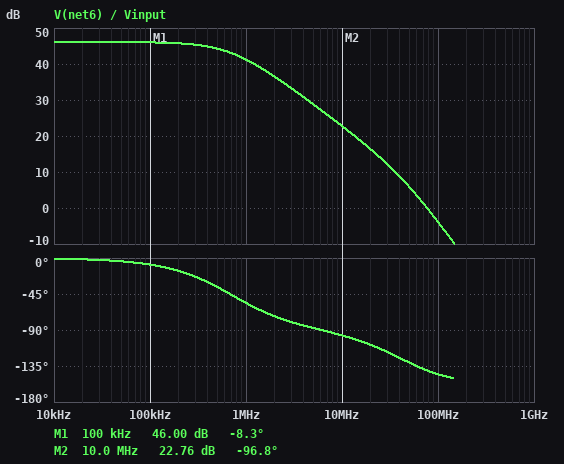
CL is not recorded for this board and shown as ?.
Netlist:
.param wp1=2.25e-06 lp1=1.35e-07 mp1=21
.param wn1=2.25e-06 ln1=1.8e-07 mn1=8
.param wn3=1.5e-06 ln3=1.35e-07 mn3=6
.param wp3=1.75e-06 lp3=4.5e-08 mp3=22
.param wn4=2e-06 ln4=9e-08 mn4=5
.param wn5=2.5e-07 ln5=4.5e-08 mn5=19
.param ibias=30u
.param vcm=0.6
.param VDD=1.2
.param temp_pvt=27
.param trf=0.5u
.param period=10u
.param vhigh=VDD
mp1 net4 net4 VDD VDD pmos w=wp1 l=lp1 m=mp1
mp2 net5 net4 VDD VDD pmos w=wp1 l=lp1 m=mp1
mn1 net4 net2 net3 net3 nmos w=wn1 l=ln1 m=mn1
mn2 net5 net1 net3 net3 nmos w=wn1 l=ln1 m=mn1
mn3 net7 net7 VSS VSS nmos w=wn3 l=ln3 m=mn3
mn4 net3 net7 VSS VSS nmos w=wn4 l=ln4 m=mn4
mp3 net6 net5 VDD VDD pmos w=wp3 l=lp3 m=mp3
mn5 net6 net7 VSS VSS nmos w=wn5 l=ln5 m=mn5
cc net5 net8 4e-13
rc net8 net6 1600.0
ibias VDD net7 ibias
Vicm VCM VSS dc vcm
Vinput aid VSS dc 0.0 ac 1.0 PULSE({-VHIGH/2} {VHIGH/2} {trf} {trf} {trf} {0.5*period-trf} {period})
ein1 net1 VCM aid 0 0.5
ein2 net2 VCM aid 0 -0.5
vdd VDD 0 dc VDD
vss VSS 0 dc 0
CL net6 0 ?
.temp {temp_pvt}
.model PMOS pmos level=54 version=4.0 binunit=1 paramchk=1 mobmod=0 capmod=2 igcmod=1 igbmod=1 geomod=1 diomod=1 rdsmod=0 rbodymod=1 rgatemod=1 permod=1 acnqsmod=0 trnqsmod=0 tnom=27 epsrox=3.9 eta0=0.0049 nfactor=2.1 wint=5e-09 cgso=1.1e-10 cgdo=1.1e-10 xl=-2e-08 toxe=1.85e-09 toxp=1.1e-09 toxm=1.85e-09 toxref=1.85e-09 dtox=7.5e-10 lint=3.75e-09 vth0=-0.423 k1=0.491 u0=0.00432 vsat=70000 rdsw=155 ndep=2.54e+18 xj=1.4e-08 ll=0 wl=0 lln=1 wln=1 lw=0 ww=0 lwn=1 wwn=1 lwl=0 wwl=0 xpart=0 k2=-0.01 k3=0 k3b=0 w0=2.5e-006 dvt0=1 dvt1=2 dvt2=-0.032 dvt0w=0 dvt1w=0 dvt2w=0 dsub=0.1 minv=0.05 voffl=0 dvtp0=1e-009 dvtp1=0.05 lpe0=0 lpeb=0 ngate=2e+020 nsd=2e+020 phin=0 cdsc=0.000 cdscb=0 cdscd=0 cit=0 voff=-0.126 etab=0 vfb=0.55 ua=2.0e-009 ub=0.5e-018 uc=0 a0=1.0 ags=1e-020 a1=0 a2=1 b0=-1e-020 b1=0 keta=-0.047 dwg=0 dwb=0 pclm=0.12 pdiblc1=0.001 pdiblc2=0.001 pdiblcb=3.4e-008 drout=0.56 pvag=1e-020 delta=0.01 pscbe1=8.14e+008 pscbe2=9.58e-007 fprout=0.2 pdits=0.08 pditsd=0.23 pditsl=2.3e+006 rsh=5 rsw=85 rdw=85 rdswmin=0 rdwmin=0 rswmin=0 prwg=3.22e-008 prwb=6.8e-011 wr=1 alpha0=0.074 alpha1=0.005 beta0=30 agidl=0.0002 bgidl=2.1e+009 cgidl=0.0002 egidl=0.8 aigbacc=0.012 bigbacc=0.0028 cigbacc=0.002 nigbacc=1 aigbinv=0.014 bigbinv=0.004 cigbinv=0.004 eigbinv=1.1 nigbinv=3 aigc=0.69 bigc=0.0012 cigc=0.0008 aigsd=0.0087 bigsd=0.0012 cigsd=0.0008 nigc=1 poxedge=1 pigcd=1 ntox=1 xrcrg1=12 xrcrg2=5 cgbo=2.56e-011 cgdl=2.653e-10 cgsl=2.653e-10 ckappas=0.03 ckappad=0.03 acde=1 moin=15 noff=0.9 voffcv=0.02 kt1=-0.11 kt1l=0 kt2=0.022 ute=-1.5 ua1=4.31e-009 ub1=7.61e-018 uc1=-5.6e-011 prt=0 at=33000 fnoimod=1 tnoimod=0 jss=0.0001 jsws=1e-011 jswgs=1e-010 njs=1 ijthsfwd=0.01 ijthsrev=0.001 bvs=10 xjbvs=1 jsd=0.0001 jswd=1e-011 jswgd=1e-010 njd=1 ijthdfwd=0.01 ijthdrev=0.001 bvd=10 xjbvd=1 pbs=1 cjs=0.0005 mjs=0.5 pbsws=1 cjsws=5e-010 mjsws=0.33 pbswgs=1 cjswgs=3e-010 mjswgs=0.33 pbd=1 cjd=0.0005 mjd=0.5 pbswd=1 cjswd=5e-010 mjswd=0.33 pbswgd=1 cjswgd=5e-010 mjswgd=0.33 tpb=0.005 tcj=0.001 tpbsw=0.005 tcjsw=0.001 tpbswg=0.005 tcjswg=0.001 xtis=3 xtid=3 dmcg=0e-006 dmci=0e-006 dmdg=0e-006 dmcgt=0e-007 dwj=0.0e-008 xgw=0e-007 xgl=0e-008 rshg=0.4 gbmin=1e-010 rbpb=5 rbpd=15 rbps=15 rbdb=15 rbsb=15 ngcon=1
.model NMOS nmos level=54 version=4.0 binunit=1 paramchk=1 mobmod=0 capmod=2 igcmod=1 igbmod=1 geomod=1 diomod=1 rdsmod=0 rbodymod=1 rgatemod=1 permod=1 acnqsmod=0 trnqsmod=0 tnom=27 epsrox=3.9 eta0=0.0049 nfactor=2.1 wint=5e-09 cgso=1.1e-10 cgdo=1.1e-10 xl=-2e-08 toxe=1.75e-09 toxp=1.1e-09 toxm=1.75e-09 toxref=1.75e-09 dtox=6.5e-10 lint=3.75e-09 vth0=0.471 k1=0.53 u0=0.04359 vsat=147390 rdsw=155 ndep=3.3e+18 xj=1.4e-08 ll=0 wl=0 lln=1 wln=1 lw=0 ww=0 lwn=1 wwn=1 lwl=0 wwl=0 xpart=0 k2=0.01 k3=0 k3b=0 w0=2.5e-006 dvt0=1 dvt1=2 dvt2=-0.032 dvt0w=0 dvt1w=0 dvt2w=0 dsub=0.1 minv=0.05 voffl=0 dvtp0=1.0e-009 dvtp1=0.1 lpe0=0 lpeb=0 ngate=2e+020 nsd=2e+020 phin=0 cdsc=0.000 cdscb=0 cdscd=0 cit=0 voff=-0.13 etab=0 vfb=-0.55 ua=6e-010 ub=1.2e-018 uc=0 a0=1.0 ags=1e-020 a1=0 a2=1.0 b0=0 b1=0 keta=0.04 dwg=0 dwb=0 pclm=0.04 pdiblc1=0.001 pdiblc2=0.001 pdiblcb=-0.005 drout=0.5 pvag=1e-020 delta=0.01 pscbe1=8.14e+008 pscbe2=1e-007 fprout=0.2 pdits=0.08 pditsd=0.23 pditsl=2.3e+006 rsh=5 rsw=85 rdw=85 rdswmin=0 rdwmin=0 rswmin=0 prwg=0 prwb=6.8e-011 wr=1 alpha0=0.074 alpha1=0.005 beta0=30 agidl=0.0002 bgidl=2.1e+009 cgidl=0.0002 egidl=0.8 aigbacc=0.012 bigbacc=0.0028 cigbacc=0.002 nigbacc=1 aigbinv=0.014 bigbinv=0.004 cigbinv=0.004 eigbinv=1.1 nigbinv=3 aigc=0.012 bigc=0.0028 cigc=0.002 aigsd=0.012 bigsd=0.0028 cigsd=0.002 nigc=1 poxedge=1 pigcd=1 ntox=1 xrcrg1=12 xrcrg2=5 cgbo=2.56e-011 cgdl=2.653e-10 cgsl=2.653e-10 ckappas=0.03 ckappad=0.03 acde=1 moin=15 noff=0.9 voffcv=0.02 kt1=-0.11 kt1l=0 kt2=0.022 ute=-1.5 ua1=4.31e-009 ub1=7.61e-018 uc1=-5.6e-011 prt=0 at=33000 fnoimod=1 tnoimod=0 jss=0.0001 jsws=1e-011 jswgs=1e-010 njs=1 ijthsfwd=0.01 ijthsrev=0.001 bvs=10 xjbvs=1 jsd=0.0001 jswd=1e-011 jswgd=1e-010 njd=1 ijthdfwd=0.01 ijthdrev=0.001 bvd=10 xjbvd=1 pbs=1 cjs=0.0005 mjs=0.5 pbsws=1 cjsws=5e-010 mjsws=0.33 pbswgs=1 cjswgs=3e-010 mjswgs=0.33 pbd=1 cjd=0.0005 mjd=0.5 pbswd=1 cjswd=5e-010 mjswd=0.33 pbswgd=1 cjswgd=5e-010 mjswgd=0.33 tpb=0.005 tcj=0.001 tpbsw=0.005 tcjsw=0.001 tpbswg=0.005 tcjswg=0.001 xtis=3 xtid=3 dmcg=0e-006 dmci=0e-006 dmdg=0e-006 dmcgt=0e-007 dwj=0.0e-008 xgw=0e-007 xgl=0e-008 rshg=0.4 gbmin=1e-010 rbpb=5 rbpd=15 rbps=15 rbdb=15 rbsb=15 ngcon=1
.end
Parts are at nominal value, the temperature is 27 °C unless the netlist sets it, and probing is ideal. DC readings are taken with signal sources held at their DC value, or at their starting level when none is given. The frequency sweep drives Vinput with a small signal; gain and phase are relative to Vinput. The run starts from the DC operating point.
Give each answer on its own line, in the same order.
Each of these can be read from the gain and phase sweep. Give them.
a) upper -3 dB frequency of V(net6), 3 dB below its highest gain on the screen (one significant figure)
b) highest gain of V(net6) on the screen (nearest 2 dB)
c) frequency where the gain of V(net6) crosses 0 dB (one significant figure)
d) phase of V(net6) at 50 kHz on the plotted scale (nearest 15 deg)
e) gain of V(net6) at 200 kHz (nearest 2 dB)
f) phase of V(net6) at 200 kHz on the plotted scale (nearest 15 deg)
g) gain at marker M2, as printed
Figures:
700 kHz
46 dB
80 MHz
0 deg
46 dB
-15 deg
22.76 dB
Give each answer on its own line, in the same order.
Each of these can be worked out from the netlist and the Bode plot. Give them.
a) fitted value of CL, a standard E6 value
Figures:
33 pF
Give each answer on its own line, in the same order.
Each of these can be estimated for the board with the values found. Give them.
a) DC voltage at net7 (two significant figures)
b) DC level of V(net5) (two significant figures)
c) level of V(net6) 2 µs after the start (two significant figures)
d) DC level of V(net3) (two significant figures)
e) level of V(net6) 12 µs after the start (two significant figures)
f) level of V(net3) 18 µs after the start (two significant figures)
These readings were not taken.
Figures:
420 mV
780 mV
1.2 V
200 mV
1.2 V
460 mV
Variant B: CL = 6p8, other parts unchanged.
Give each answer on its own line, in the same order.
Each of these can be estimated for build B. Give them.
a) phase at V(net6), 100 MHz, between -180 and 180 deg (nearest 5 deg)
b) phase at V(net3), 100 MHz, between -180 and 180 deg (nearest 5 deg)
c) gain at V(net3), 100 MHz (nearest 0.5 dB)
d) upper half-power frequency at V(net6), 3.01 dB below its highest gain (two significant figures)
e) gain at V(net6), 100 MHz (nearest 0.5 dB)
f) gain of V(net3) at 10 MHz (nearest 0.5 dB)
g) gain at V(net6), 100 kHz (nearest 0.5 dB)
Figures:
-105 deg
165 deg
-47.0 dB
720 kHz
3.0 dB
-37.5 dB
46.0 dB
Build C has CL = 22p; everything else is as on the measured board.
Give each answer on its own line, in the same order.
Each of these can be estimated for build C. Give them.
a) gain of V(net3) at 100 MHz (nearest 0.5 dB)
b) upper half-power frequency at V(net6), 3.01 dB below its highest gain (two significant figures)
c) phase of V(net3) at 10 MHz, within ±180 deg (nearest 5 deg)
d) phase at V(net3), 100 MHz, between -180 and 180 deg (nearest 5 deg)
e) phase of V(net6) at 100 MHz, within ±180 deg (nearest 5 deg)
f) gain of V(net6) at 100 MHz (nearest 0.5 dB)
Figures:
-43.0 dB
710 kHz
125 deg
160 deg
-135 deg
-1.0 dB
